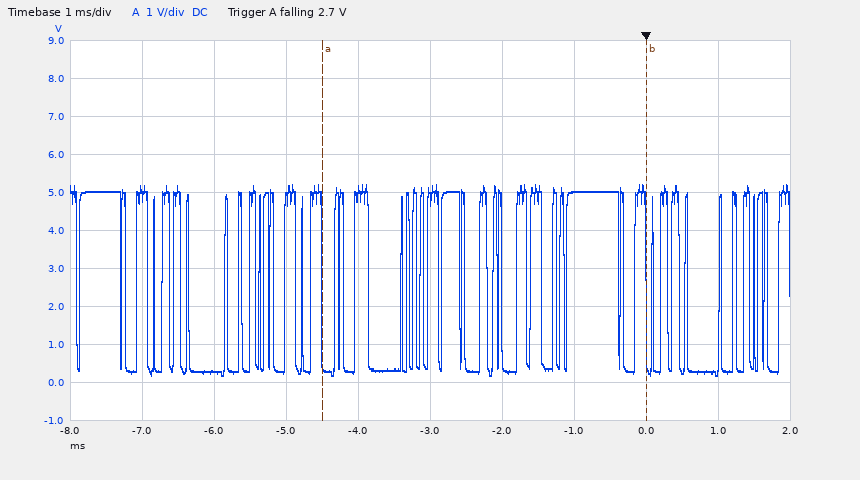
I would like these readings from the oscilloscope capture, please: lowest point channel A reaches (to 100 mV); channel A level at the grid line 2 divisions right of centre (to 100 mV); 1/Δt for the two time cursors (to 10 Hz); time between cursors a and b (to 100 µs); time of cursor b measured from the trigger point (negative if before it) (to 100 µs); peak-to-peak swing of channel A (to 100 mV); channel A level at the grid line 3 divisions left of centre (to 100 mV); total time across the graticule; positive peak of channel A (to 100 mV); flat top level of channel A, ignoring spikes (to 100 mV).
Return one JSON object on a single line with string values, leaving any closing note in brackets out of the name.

{"lowest point channel A reaches": "200 mV", "channel A level at the grid line 2 divisions right of centre": "5.0 V", "1/Δt for the two time cursors": "220 Hz", "time between cursors a and b": "4.5 ms", "time of cursor b measured from the trigger point (negative if before it)": "0.0 ms", "peak-to-peak swing of channel A": "5.0 V", "channel A level at the grid line 3 divisions left of centre": "300 mV", "total time across the graticule": "10 ms", "positive peak of channel A": "5.2 V", "flat top level of channel A, ignoring spikes": "5.0 V"}
